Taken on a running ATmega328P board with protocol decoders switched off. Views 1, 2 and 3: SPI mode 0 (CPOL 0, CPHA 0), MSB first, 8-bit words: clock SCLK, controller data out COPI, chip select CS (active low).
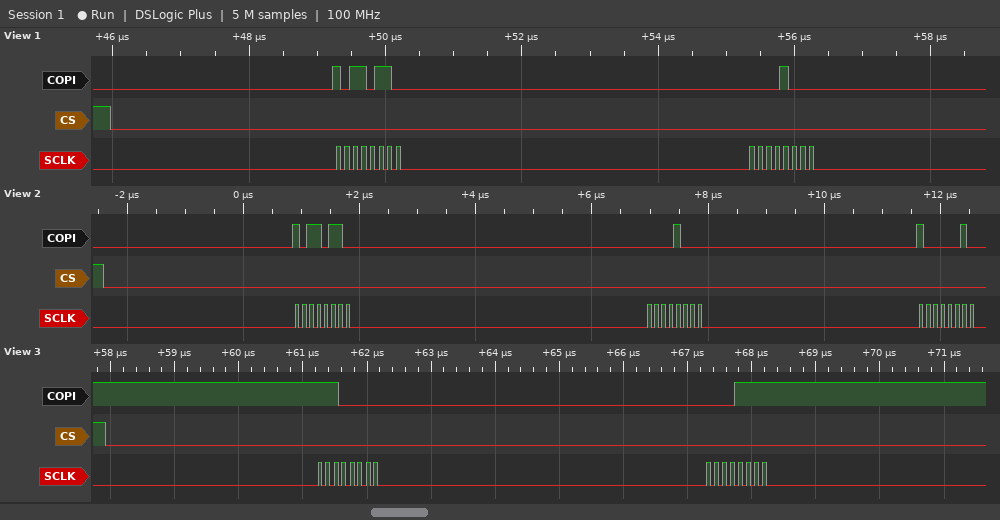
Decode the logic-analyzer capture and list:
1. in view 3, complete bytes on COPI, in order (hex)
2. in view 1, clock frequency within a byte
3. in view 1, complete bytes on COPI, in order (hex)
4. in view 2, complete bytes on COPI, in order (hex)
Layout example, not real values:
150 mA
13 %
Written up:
0xE0 0x0F
8 MHz
B6 08
0xB6 0x08 0x82
